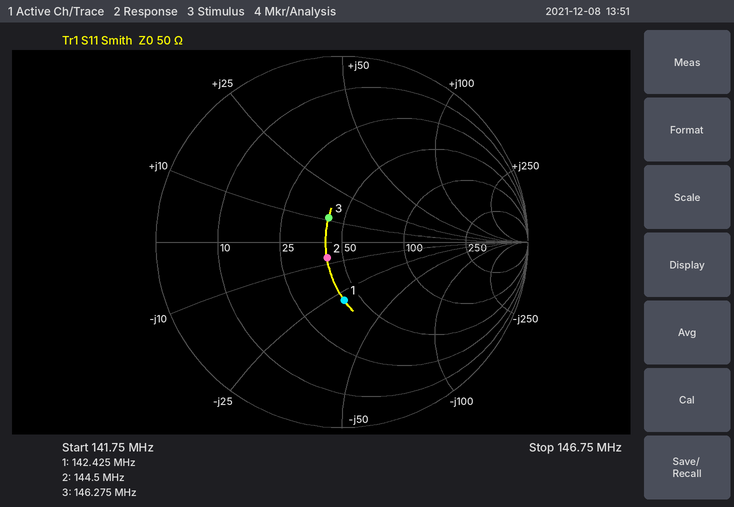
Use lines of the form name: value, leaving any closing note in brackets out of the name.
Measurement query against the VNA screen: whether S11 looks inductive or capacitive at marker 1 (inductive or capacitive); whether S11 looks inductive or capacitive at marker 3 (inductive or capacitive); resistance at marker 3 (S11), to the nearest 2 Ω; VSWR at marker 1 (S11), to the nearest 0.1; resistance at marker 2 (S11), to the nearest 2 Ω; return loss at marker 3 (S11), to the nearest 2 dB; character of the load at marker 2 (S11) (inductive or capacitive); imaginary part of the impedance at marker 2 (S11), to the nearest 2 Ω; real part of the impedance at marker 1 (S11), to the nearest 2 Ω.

whether S11 looks inductive or capacitive at marker 1: capacitive
whether S11 looks inductive or capacitive at marker 3: inductive
resistance at marker 3 (S11), to the nearest 2 Ω: 42 Ω
VSWR at marker 1 (S11), to the nearest 0.1: 1.9
resistance at marker 2 (S11), to the nearest 2 Ω: 42 Ω
return loss at marker 3 (S11), to the nearest 2 dB: 16 dB
character of the load at marker 2 (S11): capacitive
imaginary part of the impedance at marker 2 (S11), to the nearest 2 Ω: -8 Ω
real part of the impedance at marker 1 (S11), to the nearest 2 Ω: 42 Ω
